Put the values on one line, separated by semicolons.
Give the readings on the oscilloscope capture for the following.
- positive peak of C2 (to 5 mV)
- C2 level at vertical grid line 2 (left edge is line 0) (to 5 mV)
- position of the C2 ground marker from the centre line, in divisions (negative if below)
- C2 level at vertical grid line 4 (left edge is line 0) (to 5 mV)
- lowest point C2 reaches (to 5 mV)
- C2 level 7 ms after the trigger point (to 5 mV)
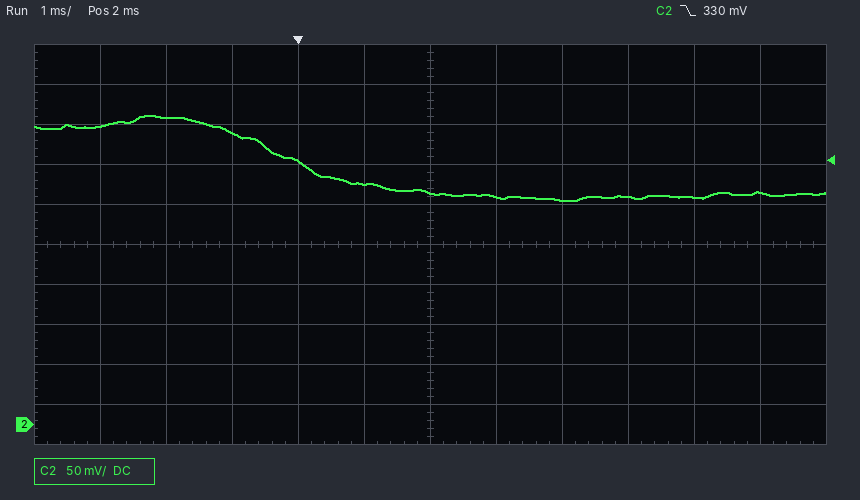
385 mV; 385 mV; -4.5 div; 330 mV; 280 mV; 290 mV
